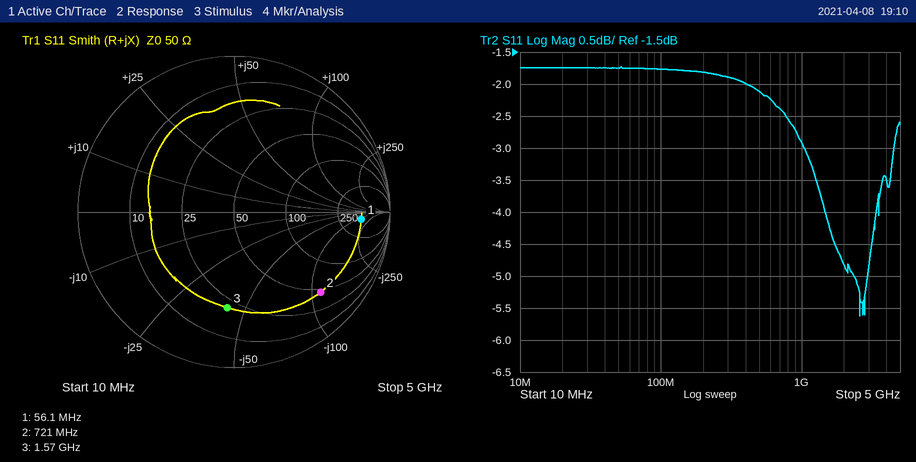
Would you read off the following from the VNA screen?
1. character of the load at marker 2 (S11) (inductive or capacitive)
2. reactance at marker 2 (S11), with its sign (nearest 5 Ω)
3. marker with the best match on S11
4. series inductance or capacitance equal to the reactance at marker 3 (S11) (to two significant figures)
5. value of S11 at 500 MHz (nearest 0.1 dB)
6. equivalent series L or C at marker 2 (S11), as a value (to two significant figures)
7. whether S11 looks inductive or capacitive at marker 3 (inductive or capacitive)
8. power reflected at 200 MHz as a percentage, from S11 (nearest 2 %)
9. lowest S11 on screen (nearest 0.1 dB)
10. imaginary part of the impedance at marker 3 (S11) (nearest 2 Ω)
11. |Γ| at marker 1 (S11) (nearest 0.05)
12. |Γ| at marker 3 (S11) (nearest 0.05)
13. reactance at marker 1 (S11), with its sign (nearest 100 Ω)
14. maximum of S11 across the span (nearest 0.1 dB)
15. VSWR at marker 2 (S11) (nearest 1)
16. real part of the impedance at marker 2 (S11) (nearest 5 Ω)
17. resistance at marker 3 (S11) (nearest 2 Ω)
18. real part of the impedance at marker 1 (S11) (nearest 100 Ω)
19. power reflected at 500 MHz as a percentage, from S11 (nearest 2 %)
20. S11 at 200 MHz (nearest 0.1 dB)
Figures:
capacitive
-110 Ω
marker 3
2.4 pF
-2.1 dB
2.0 pF
capacitive
66 %
-5.6 dB
-42 Ω
0.80
0.60
-100 Ω
-1.7 dB
7
45 Ω
22 Ω
500 Ω
62 %
-1.8 dB
